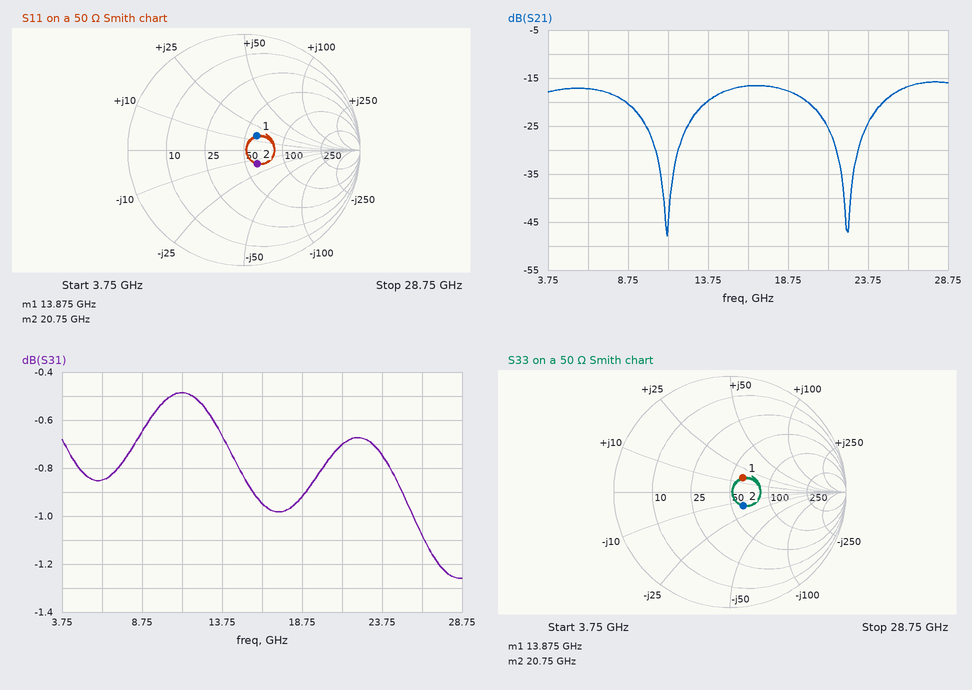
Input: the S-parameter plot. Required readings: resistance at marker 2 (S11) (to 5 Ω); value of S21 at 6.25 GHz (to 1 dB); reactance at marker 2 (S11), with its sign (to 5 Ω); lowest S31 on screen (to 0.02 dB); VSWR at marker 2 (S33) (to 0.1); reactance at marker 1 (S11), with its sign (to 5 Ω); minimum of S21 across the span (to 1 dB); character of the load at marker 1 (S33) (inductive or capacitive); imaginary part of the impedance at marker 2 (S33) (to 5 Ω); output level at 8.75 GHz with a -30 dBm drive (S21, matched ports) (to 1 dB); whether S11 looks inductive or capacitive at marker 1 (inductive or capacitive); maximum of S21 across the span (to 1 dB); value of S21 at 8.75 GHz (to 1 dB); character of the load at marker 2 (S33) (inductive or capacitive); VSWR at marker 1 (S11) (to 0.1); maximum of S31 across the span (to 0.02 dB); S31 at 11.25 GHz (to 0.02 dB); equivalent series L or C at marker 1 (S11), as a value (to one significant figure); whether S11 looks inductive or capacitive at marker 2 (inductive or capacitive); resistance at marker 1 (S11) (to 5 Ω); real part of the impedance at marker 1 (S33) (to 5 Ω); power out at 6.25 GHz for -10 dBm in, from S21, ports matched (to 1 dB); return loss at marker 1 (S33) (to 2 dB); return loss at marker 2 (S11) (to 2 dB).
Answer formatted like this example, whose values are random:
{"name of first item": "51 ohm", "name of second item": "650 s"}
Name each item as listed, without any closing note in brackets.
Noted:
{"resistance at marker 2 (S11)": "60 Ω", "value of S21 at 6.25 GHz": "-17 dB", "reactance at marker 2 (S11), with its sign": "-15 Ω", "lowest S31 on screen": "-1.26 dB", "VSWR at marker 2 (S33)": "1.4", "reactance at marker 1 (S11), with its sign": "+15 Ω", "minimum of S21 across the span": "-48 dB", "character of the load at marker 1 (S33)": "inductive", "imaginary part of the impedance at marker 2 (S33)": "-15 Ω", "output level at 8.75 GHz with a -30 dBm drive (S21, matched ports)": "-50 dBm", "whether S11 looks inductive or capacitive at marker 1": "inductive", "maximum of S21 across the span": "-16 dB", "value of S21 at 8.75 GHz": "-20 dB", "character of the load at marker 2 (S33)": "capacitive", "VSWR at marker 1 (S11)": "1.4", "maximum of S31 across the span": "-0.48 dB", "S31 at 11.25 GHz": "-0.48 dB", "equivalent series L or C at marker 1 (S11), as a value": "200 pH", "whether S11 looks inductive or capacitive at marker 2": "capacitive", "resistance at marker 1 (S11)": "60 Ω", "real part of the impedance at marker 1 (S33)": "60 Ω", "power out at 6.25 GHz for -10 dBm in, from S21, ports matched": "-27 dBm", "return loss at marker 1 (S33)": "16 dB", "return loss at marker 2 (S11)": "16 dB"}
